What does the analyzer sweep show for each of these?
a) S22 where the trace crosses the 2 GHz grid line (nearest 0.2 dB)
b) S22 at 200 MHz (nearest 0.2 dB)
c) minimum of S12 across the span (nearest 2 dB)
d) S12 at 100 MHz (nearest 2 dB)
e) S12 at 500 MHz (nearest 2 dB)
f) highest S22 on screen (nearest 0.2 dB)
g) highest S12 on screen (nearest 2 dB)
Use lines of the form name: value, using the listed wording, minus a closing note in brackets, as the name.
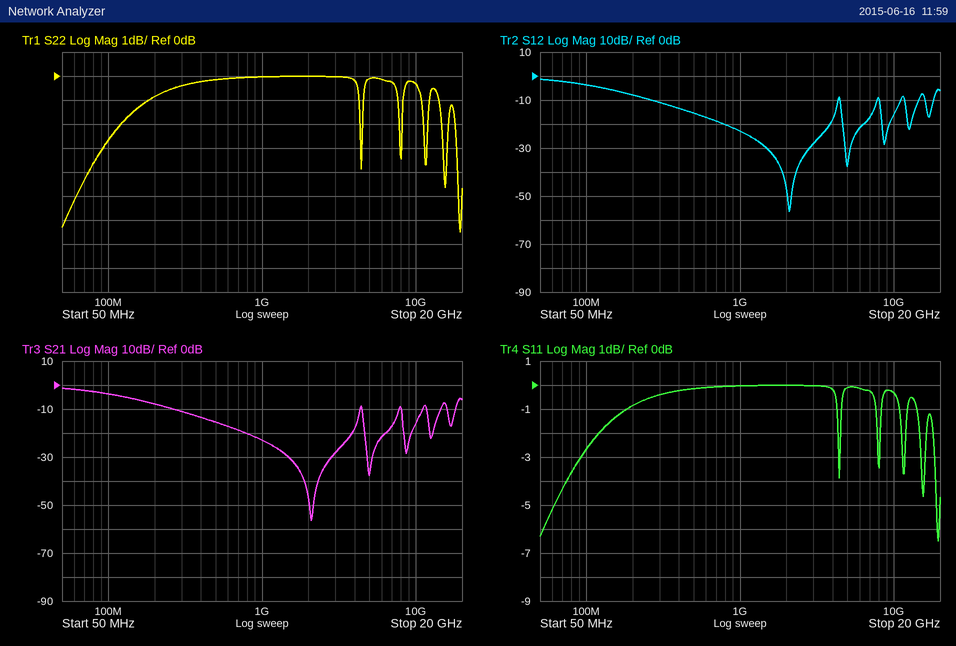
S22 where the trace crosses the 2 GHz grid line: 0.0 dB
S22 at 200 MHz: -0.8 dB
minimum of S12 across the span: -56 dB
S12 at 100 MHz: -4 dB
S12 at 500 MHz: -16 dB
highest S22 on screen: 0.0 dB
highest S12 on screen: -2 dB
